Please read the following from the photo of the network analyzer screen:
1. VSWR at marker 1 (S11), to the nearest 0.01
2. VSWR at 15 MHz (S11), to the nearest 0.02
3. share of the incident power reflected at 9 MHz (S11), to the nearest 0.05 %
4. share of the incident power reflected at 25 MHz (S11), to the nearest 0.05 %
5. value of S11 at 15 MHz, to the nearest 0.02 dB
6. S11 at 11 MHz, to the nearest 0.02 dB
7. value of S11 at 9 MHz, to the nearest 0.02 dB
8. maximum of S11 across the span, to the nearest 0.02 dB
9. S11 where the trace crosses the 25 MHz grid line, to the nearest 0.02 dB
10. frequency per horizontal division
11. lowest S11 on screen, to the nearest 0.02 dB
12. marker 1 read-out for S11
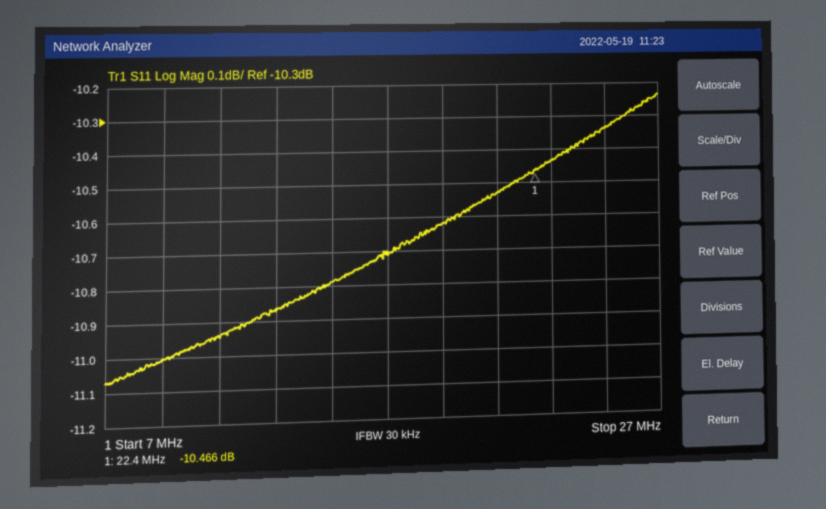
1.86
1.82
7.95 %
9.25 %
-10.78 dB
-10.94 dB
-11.00 dB
-10.24 dB
-10.34 dB
2 MHz
-11.08 dB
-10.466 dB
